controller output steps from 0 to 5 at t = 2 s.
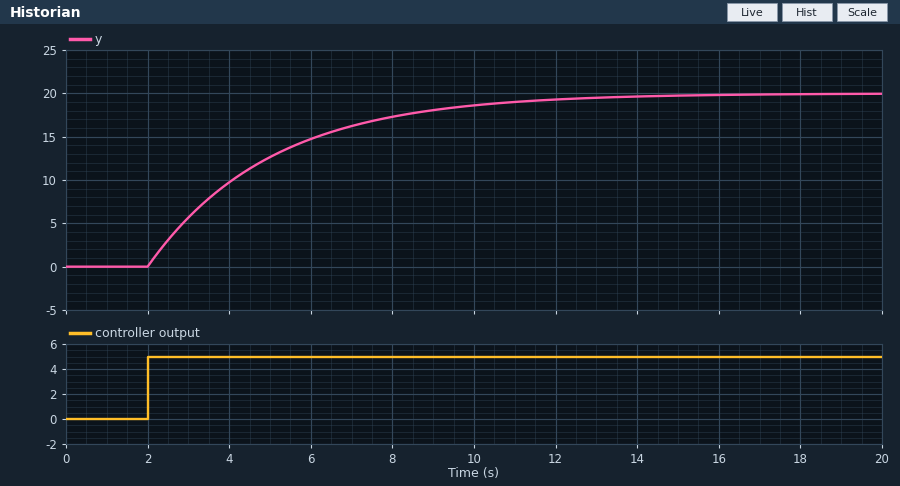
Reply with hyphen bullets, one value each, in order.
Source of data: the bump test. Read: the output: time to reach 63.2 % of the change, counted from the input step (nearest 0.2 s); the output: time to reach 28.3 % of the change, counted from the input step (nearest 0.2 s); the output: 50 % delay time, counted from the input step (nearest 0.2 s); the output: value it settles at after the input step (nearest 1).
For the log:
- 3.0 s
- 1.0 s
- 2.0 s
- 20
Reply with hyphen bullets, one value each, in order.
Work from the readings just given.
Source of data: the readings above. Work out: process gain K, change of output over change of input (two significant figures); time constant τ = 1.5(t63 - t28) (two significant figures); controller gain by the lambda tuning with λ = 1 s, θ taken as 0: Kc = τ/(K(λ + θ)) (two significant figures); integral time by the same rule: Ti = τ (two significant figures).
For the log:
- 4.0
- 3.0 s
- 0.75
- 3.0 s
